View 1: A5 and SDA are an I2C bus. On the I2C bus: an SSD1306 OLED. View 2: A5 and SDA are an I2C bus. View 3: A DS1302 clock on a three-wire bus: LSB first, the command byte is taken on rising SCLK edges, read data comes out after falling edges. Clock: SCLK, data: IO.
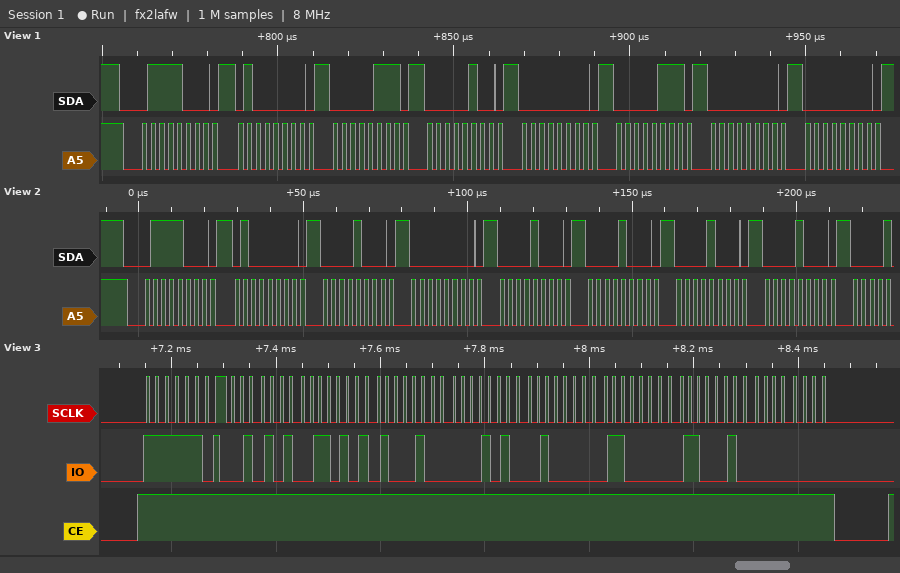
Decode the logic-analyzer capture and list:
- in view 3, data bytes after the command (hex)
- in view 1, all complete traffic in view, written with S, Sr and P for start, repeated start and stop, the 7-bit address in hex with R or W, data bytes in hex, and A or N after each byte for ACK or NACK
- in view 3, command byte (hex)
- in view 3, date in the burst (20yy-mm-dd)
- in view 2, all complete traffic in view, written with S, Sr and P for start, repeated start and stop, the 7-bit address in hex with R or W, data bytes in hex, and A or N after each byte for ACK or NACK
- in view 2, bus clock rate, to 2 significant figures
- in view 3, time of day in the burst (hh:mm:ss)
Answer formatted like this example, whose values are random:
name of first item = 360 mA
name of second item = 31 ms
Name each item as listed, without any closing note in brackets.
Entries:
in view 3, data bytes after the command = 54 56 11 28 02 03 23 00
in view 1, all complete traffic in view, written with S, Sr and P for start, repeated start and stop, the 7-bit address in hex with R or W, data bytes in hex, and A or N after each byte for ACK or NACK = S 3CW A 40 A 07 A 04 A 00 A 07 A 00 A 00 A
in view 3, command byte = 0xBF
in view 3, date in the burst = 2023-02-28
in view 2, all complete traffic in view, written with S, Sr and P for start, repeated start and stop, the 7-bit address in hex with R or W, data bytes in hex, and A or N after each byte for ACK or NACK = S 3CW A 40 A 08 A 00 A 08 A 08 A 08 A 08 A
in view 2, bus clock rate, to 2 significant figures = 400 kHz
in view 3, time of day in the burst = 11:56:54
